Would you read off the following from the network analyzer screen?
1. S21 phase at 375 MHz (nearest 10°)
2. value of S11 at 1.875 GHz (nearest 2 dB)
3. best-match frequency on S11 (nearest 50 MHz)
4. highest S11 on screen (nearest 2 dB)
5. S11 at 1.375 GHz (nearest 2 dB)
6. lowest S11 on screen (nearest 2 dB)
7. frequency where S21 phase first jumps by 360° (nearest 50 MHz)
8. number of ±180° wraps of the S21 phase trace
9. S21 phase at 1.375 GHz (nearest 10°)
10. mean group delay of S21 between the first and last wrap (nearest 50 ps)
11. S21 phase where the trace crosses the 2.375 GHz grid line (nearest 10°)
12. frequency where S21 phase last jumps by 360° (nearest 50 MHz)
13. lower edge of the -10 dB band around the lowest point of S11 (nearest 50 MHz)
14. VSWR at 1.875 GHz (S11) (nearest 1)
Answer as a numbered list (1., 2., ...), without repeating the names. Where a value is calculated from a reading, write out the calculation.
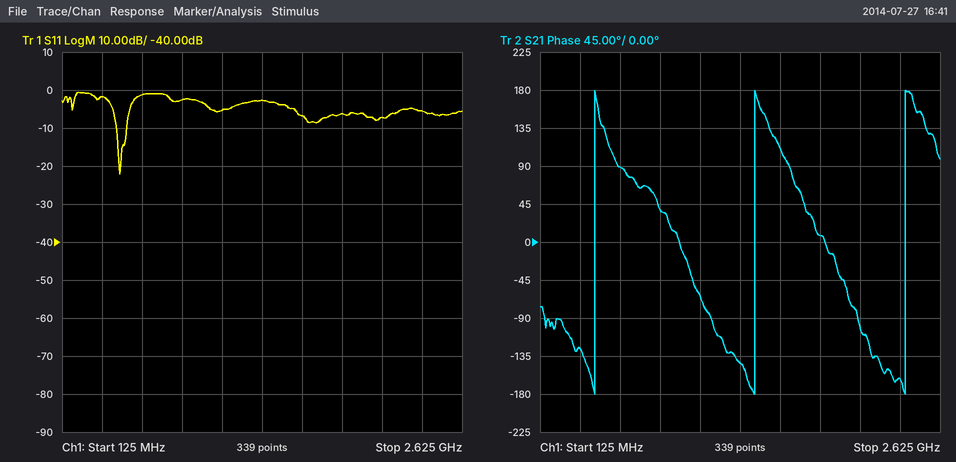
1. -130°
2. -6 dB
3. 500 MHz
4. 0 dB
5. -2 dB
6. -22 dB
7. 450 MHz
8. 3
9. -140°
10. 2 cycles / (2.40 GHz − 450 MHz) ≈ 1.03 ns, so 1.05 ns to the nearest 50 ps
11. -160°
12. 2.40 GHz
13. 450 MHz
14. |Γ| = 10^(-6/20) = 0.5012; VSWR = (1 + 0.5012)/(1 − 0.5012) ≈ 3
